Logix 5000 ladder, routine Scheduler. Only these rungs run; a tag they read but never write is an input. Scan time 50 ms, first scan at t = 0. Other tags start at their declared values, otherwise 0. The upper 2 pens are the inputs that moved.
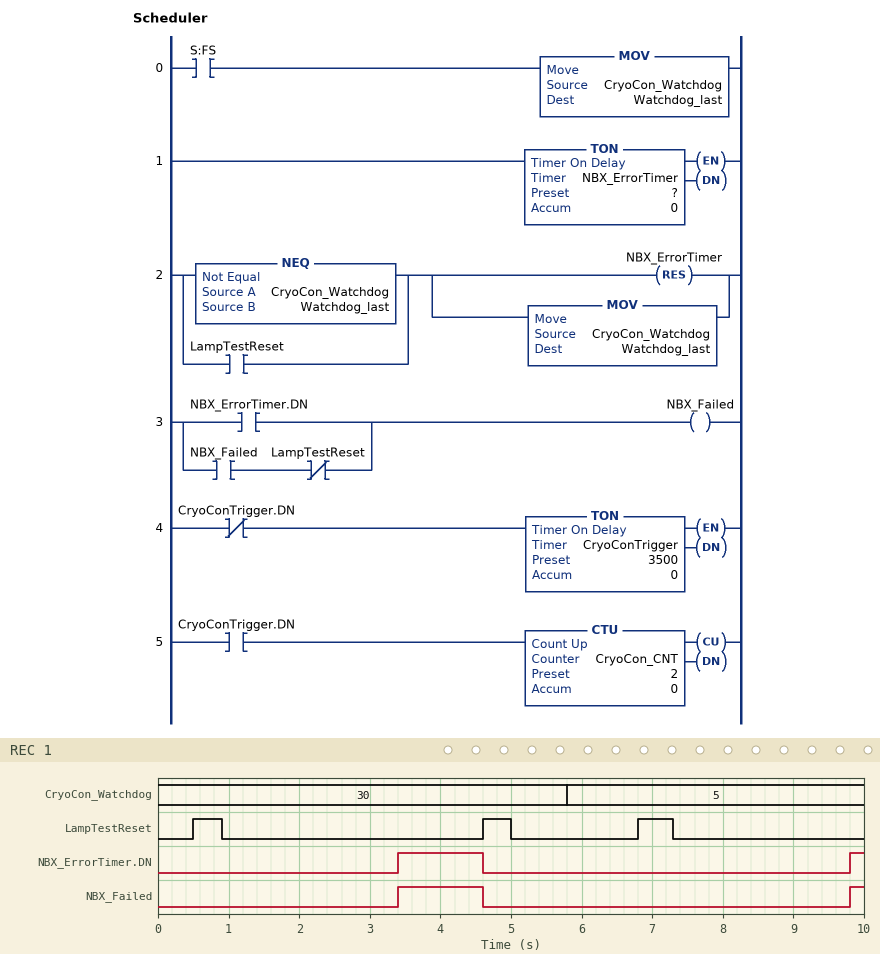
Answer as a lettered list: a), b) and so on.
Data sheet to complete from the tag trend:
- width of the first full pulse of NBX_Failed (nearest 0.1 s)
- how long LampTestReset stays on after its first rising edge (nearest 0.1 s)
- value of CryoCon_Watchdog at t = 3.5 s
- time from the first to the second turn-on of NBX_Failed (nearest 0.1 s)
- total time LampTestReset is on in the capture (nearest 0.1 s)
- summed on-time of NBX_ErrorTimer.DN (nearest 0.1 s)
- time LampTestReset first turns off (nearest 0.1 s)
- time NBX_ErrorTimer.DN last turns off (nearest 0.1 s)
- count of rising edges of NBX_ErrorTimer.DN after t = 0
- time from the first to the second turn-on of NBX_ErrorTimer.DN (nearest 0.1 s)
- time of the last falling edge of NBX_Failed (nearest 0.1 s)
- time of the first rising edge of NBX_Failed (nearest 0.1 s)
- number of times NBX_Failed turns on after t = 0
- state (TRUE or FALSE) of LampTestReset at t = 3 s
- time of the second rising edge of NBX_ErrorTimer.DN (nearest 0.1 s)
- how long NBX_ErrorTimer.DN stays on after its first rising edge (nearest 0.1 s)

a) 1.2 s
b) 0.4 s
c) 30
d) 6.4 s
e) 1.3 s
f) 1.4 s
g) 0.9 s
h) 4.6 s
i) 2
j) 6.4 s
k) 4.6 s
l) 3.4 s
m) 2
n) FALSE
o) 9.8 s
p) 1.2 s
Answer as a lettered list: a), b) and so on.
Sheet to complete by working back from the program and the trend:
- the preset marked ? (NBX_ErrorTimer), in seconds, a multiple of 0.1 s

a) 2.5 s
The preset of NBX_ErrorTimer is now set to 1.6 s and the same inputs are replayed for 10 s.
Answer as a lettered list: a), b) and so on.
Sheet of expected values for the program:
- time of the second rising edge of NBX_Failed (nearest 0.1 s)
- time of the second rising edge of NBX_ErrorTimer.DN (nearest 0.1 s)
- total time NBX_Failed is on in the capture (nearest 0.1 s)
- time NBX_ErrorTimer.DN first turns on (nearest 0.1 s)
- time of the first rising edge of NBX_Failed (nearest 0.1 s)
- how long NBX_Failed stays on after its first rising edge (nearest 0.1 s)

a) 8.9 s
b) 8.9 s
c) 3.2 s
d) 2.5 s
e) 2.5 s
f) 2.1 s
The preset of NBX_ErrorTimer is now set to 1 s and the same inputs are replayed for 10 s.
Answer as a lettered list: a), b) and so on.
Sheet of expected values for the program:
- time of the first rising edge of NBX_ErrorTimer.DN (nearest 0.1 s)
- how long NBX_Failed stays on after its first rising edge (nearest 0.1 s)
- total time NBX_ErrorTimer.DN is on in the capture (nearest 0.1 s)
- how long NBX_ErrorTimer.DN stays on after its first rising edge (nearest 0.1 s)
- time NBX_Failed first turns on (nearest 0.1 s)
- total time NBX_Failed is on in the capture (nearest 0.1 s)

a) 1.9 s
b) 2.7 s
c) 4.4 s
d) 2.7 s
e) 1.9 s
f) 4.4 s
